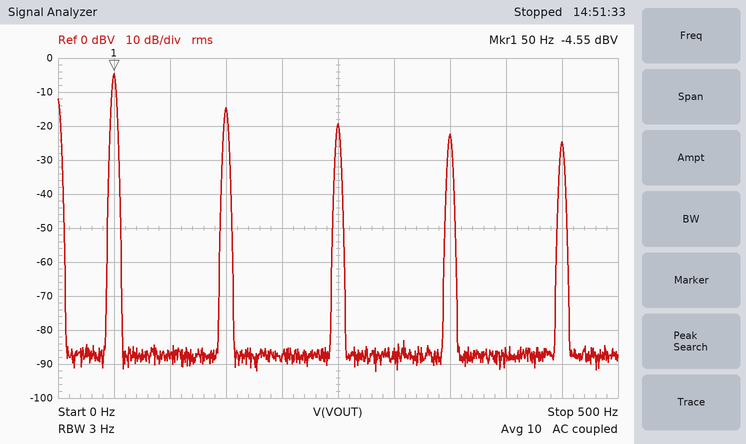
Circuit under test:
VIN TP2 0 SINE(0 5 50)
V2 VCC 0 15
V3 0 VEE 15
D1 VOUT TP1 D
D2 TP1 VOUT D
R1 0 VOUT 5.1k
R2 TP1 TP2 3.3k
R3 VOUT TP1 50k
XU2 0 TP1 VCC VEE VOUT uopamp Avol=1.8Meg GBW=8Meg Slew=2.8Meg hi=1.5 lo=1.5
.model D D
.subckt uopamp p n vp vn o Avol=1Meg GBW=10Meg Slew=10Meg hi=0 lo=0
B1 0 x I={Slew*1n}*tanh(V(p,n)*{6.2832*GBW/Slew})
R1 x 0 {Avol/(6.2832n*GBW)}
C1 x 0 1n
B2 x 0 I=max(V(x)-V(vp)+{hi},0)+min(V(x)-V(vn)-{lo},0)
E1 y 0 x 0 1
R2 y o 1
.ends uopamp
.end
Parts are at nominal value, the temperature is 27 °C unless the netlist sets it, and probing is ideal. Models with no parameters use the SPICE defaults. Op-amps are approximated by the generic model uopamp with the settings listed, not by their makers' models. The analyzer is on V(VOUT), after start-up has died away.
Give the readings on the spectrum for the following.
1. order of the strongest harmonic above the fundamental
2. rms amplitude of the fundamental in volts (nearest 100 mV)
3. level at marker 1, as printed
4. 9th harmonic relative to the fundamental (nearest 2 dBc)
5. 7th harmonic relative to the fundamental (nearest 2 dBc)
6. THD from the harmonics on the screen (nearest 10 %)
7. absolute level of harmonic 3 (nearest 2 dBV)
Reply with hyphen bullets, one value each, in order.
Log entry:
- 3
- 600 mV
- -4.55 dBV
- -20 dBc
- -18 dBc
- 40 %
- -14 dBV
